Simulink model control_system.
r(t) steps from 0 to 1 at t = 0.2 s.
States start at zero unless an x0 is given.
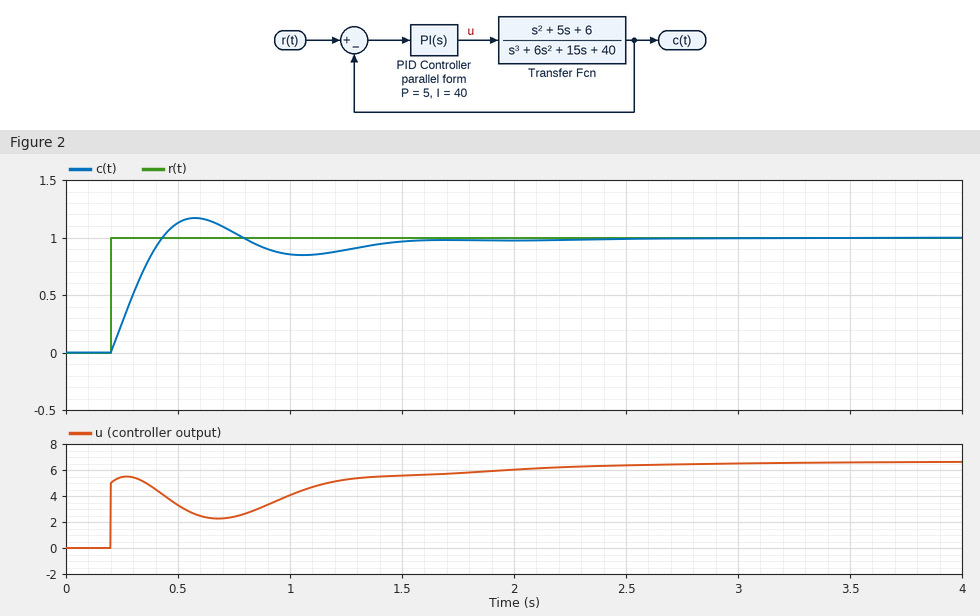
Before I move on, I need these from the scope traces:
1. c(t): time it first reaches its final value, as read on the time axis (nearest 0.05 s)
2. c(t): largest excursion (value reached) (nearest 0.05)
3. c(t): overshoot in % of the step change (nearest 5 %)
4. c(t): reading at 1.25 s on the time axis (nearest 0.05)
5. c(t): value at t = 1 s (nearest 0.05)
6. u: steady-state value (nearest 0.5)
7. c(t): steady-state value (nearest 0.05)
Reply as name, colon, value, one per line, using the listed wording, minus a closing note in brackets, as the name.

c(t): time it first reaches its final value, as read on the time axis: 0.45 s
c(t): largest excursion (value reached): 1.15
c(t): overshoot in % of the step change: 15 %
c(t): reading at 1.25 s on the time axis: 0.90
c(t): value at t = 1 s: 0.85
u: steady-state value: 6.5
c(t): steady-state value: 1.00
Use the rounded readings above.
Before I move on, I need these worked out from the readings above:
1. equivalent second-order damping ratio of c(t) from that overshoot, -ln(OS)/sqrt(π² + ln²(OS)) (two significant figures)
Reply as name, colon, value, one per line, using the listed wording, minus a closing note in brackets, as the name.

equivalent second-order damping ratio of c(t) from that overshoot, -ln(OS)/sqrt(π² + ln²(OS)): 0.52
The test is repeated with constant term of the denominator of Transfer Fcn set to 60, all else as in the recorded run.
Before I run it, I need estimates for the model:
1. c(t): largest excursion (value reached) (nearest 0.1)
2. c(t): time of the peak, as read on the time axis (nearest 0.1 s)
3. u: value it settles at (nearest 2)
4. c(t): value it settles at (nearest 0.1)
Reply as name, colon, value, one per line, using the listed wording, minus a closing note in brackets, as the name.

c(t): largest excursion (value reached): 1.1
c(t): time of the peak, as read on the time axis: 0.6 s
u: value it settles at: 10
c(t): value it settles at: 1.0
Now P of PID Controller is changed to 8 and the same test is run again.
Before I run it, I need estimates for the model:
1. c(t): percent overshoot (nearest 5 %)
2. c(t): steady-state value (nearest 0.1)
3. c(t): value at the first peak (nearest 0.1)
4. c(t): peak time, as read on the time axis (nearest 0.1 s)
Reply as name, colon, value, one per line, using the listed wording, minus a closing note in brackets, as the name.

c(t): percent overshoot: 10 %
c(t): steady-state value: 1.0
c(t): value at the first peak: 1.1
c(t): peak time, as read on the time axis: 0.5 s
